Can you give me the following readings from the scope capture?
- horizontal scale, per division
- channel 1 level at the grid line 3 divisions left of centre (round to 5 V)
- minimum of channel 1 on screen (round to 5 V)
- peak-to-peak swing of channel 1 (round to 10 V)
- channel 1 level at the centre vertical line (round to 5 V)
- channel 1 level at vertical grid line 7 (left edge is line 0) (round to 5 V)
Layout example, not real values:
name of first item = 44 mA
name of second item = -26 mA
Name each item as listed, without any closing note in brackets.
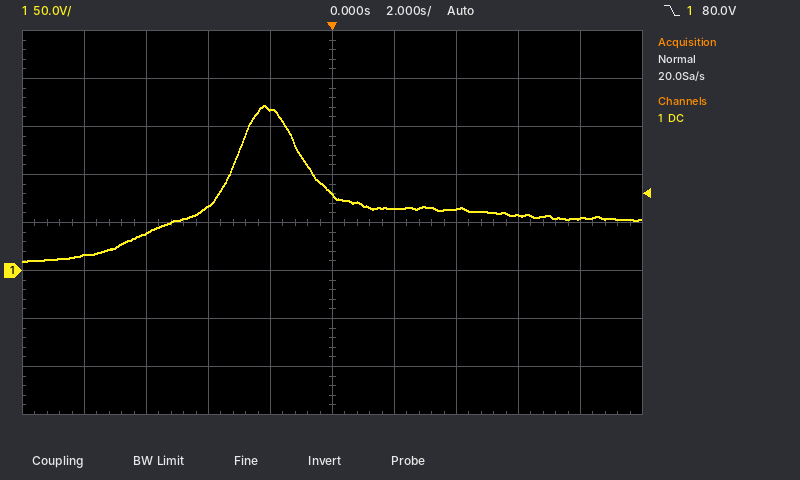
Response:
horizontal scale, per division = 2 s
channel 1 level at the grid line 3 divisions left of centre = 40 V
minimum of channel 1 on screen = 10 V
peak-to-peak swing of channel 1 = 160 V
channel 1 level at the centre vertical line = 80 V
channel 1 level at vertical grid line 7 (left edge is line 0) = 65 V
